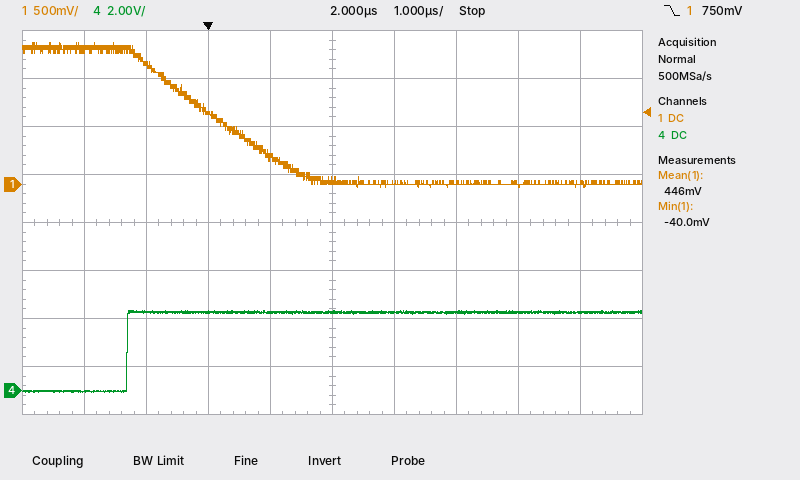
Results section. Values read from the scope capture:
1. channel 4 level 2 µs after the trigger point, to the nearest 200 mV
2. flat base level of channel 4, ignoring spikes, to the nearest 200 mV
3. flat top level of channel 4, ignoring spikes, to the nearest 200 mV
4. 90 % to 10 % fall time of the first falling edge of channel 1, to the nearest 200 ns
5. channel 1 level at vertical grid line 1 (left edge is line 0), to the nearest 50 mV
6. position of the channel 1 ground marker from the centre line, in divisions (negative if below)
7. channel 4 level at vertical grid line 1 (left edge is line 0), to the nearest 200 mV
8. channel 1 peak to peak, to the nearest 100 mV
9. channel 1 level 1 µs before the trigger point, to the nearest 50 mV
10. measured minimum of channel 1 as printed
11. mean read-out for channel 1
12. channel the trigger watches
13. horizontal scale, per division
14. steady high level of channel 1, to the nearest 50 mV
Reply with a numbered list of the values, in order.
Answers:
1. 3.2 V
2. 0.0 V
3. 3.2 V
4. 2.4 µs
5. 1.40 V
6. +0.8 div
7. 0.0 V
8. 1.50 V
9. 1.25 V
10. -40.0 mV
11. 446 mV
12. channel 1
13. 1 µs
14. 1.40 V
